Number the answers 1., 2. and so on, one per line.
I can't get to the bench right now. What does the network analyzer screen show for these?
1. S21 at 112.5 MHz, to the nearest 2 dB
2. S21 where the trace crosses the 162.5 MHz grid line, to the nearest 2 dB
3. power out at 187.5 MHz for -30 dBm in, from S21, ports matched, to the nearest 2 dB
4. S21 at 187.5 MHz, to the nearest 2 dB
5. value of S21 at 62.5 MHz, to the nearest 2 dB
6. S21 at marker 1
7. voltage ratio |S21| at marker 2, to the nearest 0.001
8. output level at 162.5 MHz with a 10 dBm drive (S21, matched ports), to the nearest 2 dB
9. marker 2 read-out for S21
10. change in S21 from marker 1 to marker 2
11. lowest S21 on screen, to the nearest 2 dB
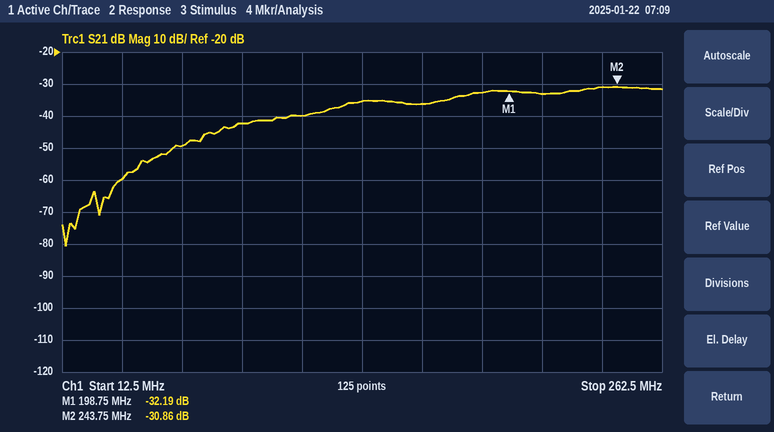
1. -40 dB
2. -36 dB
3. -62 dBm
4. -32 dB
5. -50 dB
6. -32.19 dB
7. 0.029
8. -26 dBm
9. -30.86 dB
10. 1.33 dB
11. -80 dB
